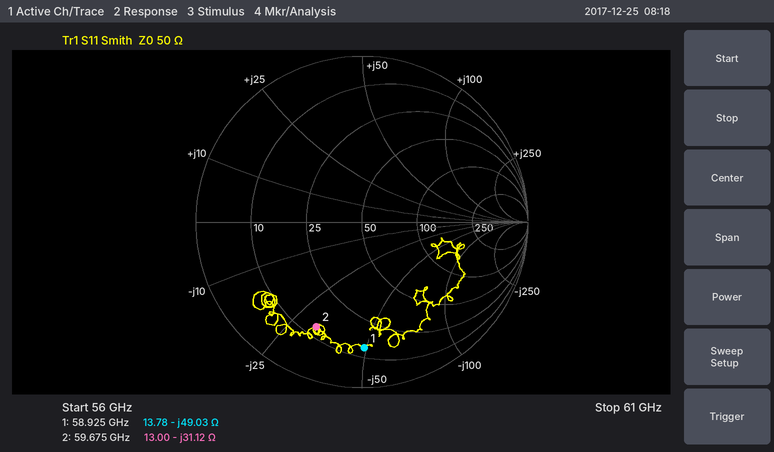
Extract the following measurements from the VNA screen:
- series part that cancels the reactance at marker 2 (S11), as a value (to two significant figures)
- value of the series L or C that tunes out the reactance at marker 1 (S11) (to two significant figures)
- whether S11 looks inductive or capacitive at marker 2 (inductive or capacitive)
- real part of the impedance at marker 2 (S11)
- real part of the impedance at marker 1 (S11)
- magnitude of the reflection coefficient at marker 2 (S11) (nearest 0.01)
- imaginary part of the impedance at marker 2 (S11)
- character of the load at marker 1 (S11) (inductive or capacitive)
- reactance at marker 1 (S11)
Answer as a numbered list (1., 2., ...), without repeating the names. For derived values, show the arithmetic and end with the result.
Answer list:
1. L = 31.12 Ω/(2π × 59.675 GHz) ≈ 83 pH
2. L = 49.03 Ω/(2π × 58.925 GHz) ≈ 132 pH, so 130 pH to two significant figures
3. capacitive
4. 13.00 Ω
5. 13.78 Ω
6. 0.69
7. -31.12 Ω
8. capacitive
9. -49.03 Ω
